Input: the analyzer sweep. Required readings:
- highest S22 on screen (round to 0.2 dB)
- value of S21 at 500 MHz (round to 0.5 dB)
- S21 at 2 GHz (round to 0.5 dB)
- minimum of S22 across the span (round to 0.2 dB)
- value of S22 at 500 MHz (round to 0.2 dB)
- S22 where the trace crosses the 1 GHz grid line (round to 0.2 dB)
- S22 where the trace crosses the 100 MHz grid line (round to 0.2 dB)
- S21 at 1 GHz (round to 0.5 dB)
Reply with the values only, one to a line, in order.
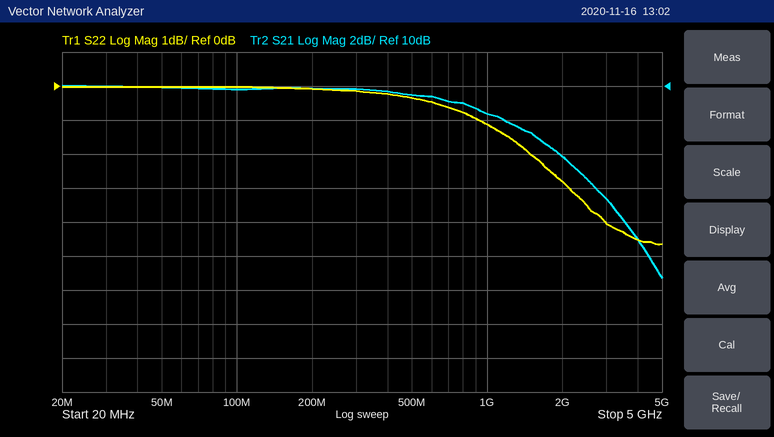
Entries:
0.0 dB
9.5 dB
6.0 dB
-4.6 dB
-0.4 dB
-1.2 dB
0.0 dB
8.5 dB
